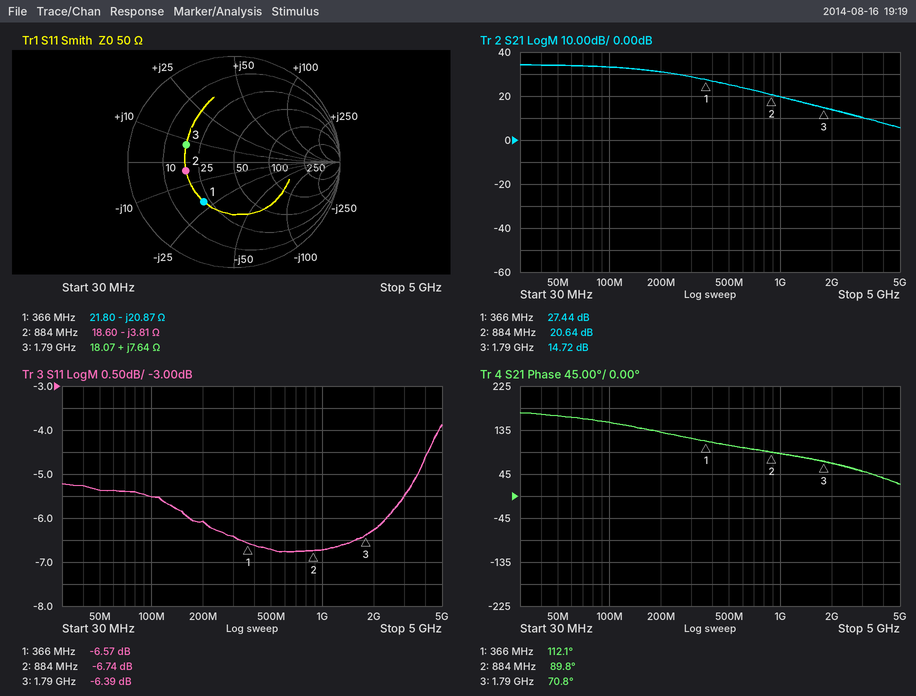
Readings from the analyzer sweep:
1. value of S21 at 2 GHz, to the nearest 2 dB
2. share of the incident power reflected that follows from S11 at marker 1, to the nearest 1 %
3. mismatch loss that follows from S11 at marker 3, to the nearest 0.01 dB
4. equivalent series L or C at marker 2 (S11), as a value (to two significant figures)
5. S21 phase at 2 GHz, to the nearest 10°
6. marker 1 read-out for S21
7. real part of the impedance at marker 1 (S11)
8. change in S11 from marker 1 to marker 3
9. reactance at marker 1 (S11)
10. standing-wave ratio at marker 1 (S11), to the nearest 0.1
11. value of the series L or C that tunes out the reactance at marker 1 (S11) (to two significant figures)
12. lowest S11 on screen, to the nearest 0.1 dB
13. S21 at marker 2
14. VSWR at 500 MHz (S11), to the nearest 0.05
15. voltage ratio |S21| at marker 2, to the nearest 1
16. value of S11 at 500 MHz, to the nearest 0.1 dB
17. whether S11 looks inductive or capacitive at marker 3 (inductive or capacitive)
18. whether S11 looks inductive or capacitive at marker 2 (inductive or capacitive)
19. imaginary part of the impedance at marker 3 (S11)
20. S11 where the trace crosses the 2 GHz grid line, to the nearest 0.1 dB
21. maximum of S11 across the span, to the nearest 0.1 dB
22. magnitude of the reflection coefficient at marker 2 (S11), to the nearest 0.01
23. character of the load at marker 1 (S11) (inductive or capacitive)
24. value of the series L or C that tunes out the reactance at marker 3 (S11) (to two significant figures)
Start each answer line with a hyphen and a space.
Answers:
- 14 dB
- 22 %
- 1.13 dB
- 47 pF
- 70°
- 27.44 dB
- 21.80 Ω
- 0.18 dB
- -20.87 Ω
- 2.8
- 9.1 nH
- -6.8 dB
- 20.64 dB
- 2.70
- 11
- -6.7 dB
- inductive
- capacitive
- +7.64 Ω
- -6.3 dB
- -3.9 dB
- 0.46
- capacitive
- 12 pF
